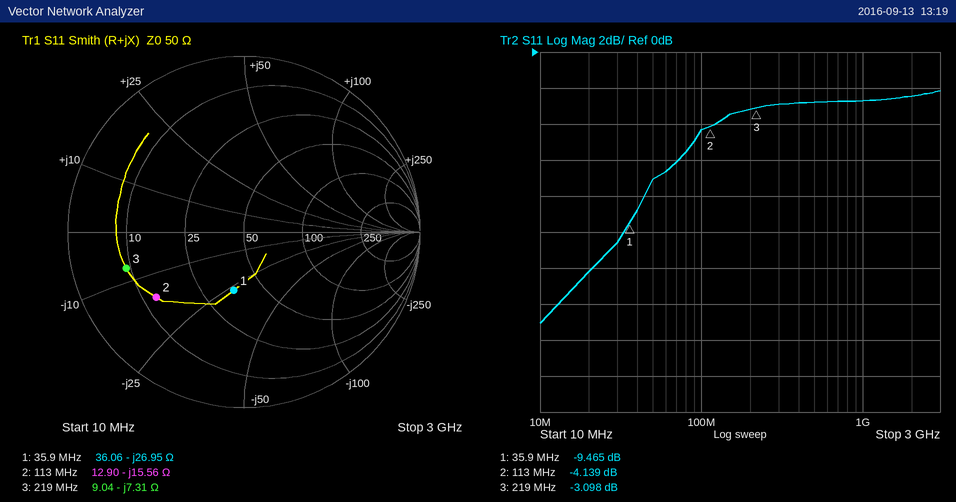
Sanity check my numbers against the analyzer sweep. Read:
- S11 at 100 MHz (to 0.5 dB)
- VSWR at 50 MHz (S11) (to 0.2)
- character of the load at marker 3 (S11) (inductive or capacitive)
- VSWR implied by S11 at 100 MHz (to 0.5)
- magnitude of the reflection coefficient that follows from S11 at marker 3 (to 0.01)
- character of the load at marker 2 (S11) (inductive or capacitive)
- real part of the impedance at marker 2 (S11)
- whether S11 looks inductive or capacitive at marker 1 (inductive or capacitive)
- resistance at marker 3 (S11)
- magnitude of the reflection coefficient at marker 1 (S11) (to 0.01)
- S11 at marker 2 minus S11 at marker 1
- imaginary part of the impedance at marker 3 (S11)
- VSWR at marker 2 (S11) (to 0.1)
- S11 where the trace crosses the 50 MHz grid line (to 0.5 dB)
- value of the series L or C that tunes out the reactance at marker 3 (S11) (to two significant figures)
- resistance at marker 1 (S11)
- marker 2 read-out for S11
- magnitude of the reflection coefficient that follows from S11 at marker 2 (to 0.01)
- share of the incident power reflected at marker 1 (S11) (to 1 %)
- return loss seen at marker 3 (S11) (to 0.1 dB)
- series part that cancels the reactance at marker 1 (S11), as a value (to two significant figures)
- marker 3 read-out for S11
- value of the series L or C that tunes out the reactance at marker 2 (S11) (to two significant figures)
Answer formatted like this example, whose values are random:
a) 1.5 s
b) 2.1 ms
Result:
a) -4.5 dB
b) 2.6
c) capacitive
d) 4.0
e) 0.70
f) capacitive
g) 12.90 Ω
h) capacitive
i) 9.04 Ω
j) 0.34
k) 5.326 dB
l) -7.31 Ω
m) 4.3
n) -7.0 dB
o) 5.3 nH
p) 36.06 Ω
q) -4.139 dB
r) 0.62
s) 11 %
t) 3.1 dB
u) 120 nH
v) -3.098 dB
w) 22 nH
